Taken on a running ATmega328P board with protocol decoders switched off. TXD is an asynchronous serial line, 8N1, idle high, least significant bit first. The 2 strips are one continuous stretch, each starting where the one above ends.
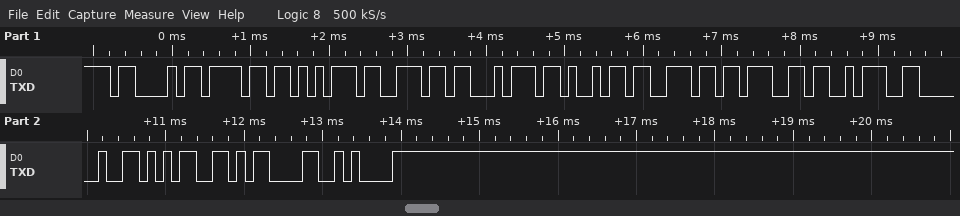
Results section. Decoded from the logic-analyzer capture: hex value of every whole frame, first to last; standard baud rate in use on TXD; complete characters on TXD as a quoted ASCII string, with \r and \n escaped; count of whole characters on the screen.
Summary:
43 6F 75 6E 74 69 6E 67 3A 20 35 0D 0A
9600 baud
"Counting: 5\r\n"
13
